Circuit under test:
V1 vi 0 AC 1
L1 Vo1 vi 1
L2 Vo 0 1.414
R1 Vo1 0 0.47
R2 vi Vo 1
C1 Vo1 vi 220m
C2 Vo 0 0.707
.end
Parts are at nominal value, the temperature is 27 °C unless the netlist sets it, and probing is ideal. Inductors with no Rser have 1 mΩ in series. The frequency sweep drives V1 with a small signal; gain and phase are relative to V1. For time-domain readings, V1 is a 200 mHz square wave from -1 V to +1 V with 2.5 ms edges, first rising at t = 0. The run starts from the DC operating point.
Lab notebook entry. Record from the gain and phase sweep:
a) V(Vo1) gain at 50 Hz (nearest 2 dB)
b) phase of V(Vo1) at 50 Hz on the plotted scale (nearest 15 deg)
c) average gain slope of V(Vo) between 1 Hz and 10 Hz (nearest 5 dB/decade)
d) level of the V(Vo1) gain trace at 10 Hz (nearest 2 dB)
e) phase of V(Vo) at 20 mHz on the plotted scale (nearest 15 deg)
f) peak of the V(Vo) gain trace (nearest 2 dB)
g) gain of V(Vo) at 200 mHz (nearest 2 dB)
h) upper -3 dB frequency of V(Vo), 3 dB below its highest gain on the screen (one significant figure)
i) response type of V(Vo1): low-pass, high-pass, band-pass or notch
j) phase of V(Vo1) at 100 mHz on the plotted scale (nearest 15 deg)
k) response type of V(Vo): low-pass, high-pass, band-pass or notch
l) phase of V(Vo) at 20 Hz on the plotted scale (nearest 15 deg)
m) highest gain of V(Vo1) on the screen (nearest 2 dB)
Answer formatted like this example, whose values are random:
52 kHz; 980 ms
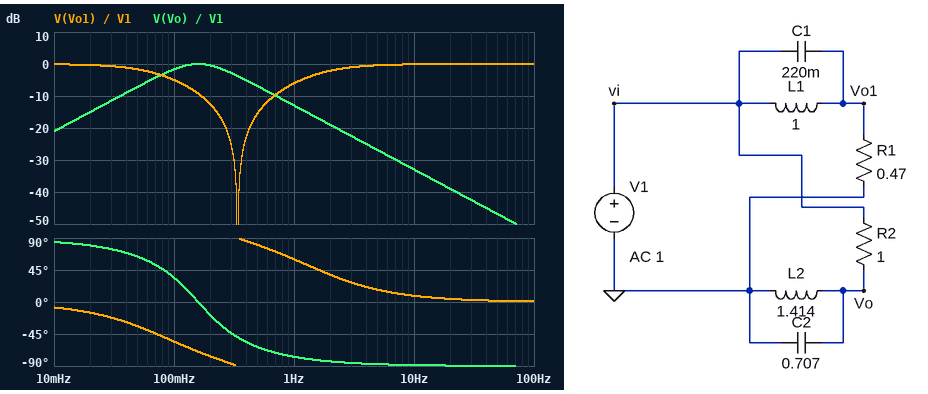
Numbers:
0 dB; 0 deg; -20 dB/decade; 0 dB; 75 deg; 0 dB; 0 dB; 300 mHz; notch; -60 deg; band-pass; -90 deg; 0 dB
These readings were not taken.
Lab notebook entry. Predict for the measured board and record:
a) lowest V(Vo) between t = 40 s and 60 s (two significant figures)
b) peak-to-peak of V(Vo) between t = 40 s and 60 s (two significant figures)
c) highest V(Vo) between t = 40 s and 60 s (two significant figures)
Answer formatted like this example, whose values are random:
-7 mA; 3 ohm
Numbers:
-1.1 V; 2.2 V; 1.1 V
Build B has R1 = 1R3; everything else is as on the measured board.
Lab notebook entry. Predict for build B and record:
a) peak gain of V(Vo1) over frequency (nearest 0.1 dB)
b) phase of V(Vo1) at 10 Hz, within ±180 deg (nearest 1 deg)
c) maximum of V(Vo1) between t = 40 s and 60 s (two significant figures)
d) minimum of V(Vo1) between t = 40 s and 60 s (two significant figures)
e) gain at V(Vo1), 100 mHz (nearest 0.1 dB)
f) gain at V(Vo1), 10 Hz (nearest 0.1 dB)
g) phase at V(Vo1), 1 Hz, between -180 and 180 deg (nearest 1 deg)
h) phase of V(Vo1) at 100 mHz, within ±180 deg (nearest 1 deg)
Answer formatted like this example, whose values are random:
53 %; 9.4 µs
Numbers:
0 dB; 3 deg; 1.0 V; -1.0 V; -1.1 dB; 0 dB; 32 deg; -28 deg
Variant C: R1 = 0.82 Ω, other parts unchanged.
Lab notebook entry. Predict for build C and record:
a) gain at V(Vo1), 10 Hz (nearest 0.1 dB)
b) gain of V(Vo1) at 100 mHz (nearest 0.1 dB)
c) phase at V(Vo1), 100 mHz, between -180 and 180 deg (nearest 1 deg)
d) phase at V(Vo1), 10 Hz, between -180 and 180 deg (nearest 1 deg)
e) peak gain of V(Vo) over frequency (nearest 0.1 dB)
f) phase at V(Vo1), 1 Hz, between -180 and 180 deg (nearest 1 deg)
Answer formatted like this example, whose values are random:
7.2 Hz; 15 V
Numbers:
0 dB; -2.3 dB; -40 deg; 5 deg; 0 dB; 45 deg
